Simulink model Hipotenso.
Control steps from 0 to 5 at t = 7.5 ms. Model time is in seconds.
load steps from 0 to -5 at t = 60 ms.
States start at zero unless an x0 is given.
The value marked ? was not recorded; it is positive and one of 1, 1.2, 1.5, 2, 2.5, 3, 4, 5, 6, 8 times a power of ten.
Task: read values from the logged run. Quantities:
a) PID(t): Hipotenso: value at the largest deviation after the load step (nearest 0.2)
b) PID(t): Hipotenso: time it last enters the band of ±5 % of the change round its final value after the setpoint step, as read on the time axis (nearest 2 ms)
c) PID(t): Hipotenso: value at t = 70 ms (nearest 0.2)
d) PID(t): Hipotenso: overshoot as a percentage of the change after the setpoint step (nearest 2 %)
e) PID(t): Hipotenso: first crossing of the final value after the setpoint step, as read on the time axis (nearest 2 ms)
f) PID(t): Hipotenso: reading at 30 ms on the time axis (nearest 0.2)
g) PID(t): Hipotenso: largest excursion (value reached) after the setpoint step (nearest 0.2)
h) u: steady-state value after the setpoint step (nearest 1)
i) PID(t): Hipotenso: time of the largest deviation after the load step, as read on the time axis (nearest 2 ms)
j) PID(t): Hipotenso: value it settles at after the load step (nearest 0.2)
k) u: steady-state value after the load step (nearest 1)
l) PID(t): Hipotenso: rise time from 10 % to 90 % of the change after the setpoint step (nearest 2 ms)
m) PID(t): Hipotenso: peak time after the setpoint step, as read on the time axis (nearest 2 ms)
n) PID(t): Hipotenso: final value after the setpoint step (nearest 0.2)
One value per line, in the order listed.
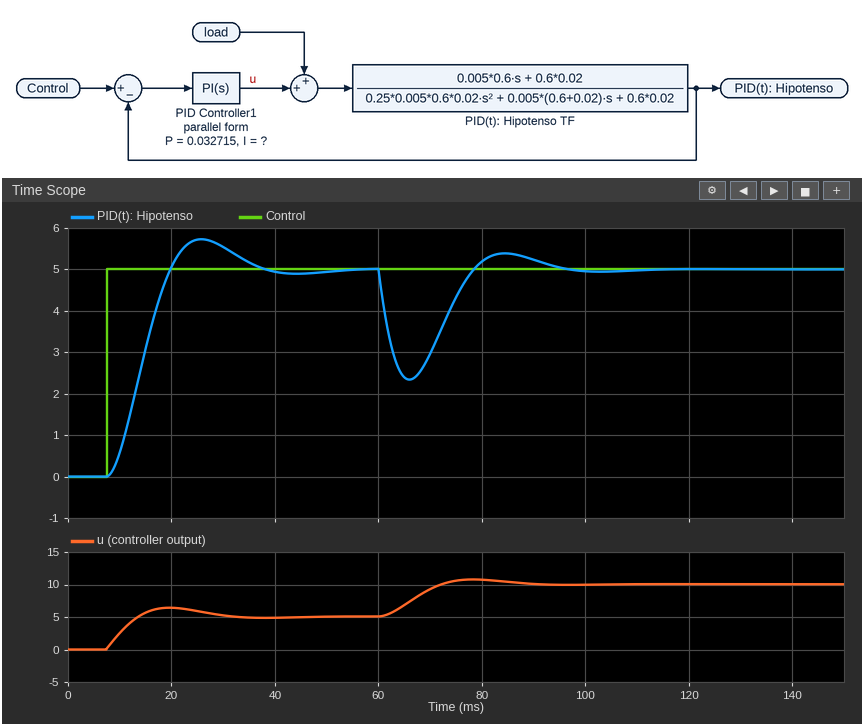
2.4
34 ms
3.0
14 %
20 ms
5.6
5.8
5
66 ms
5.0
10
8 ms
26 ms
5.0
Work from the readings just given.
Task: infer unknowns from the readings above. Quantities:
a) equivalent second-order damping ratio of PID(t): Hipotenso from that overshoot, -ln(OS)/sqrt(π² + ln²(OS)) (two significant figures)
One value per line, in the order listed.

0.53
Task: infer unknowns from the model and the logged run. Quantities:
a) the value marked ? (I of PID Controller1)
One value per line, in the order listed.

200
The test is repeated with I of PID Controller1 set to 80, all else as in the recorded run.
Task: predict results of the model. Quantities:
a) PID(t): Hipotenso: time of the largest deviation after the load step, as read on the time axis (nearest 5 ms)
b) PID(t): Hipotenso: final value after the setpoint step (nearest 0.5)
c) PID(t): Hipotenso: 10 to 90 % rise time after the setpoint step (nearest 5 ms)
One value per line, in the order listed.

70 ms
5.0
20 ms
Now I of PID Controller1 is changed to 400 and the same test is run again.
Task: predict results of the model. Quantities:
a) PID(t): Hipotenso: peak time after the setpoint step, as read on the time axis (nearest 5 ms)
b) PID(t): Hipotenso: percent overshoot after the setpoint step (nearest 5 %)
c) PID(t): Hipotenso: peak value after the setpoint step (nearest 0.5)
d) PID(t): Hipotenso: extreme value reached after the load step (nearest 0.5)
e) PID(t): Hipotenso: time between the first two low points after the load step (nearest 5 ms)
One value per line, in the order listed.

20 ms
30 %
6.5
3.0
25 ms
